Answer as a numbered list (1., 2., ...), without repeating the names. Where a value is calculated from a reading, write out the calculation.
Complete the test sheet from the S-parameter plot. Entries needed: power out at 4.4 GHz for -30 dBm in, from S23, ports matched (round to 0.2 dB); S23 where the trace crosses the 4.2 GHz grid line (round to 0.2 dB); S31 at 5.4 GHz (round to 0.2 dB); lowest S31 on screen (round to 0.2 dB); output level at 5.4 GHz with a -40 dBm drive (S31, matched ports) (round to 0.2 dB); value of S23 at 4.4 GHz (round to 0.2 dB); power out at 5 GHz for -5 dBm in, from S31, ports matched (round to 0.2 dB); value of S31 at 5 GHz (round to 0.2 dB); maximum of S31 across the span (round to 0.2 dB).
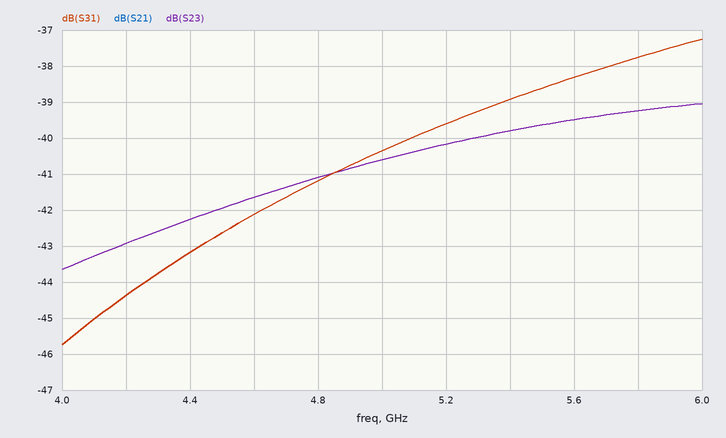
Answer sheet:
1. -30 dBm + (-42.2 dB) = -72.2 dBm
2. -43.0 dB
3. -39.0 dB
4. -45.8 dB
5. -40 dBm + (-39.0 dB) = -79.0 dBm
6. -42.2 dB
7. -5 dBm + (-40.4 dB) = -45.4 dBm
8. -40.4 dB
9. -37.2 dB
